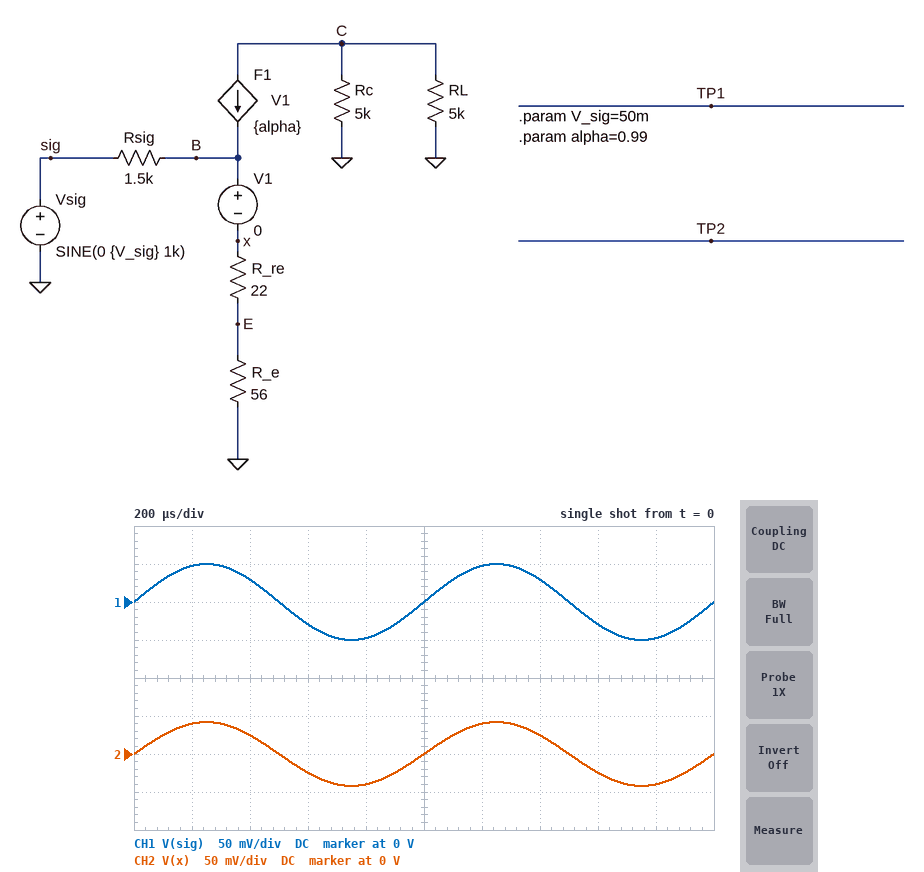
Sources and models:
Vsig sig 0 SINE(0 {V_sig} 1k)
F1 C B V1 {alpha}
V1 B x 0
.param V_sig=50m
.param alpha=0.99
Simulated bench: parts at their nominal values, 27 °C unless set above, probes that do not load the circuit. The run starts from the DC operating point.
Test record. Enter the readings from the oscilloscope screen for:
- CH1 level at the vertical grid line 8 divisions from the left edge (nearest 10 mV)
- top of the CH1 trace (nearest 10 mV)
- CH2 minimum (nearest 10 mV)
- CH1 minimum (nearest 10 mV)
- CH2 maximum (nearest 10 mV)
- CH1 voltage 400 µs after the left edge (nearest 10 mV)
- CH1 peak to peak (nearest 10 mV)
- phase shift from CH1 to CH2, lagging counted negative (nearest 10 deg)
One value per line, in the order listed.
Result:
-30 mV
50 mV
-40 mV
-50 mV
40 mV
30 mV
100 mV
0 deg
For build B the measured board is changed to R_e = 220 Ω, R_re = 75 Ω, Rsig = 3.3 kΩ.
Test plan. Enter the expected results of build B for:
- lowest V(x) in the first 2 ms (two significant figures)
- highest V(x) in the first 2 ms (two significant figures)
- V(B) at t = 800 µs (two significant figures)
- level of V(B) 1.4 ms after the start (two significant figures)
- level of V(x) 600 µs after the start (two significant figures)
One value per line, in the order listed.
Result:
-45 mV
45 mV
-43 mV
26 mV
-26 mV
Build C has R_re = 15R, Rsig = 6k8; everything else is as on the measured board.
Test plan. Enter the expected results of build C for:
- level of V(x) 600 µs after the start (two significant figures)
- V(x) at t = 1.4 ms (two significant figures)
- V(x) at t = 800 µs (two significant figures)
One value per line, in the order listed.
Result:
-15 mV
15 mV
-24 mV
